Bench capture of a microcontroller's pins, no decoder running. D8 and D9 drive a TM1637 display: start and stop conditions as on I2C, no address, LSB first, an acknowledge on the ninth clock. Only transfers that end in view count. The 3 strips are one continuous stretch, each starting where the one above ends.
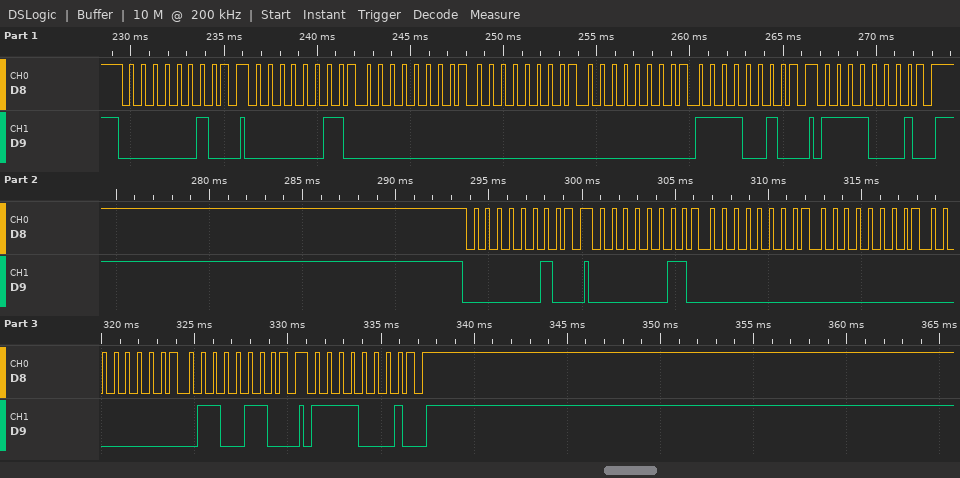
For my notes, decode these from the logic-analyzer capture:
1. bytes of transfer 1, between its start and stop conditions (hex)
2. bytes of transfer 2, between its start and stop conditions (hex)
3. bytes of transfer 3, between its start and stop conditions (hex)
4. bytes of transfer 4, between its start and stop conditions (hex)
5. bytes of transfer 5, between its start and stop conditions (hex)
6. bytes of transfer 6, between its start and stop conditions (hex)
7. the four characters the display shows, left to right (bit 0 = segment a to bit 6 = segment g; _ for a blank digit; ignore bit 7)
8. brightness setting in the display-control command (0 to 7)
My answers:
40
C0 00 00 00 4F
8F
40
C0 00 00 00 66
8F
___4
7
